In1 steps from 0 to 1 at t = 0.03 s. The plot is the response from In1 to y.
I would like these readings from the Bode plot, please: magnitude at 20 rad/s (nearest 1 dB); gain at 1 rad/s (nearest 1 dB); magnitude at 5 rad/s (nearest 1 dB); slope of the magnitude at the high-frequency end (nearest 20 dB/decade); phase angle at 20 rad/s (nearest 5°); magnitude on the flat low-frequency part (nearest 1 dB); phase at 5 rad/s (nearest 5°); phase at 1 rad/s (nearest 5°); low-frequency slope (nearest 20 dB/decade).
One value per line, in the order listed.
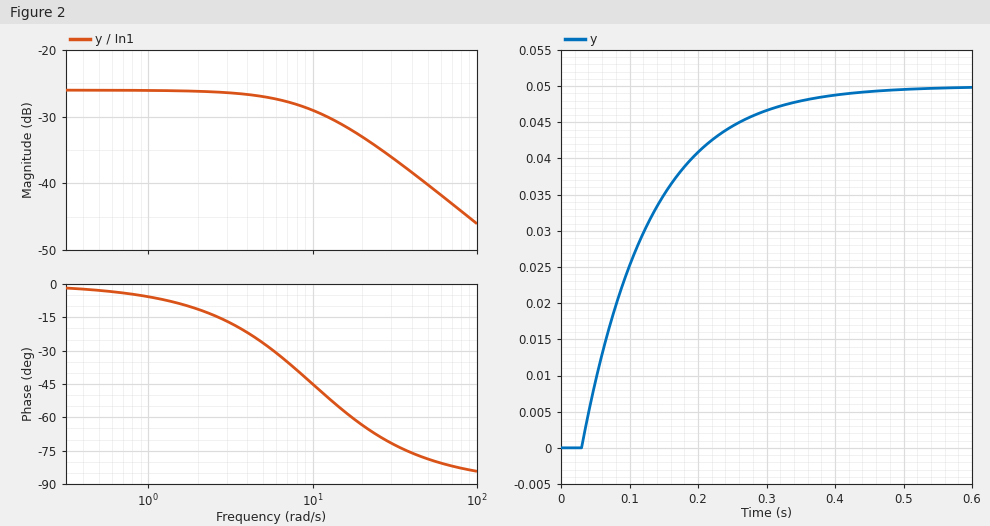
-33 dB
-26 dB
-27 dB
-20 dB/decade
-65°
-26 dB
-25°
-5°
0 dB/decade
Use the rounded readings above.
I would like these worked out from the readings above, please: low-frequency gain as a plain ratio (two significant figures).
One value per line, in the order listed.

0.050
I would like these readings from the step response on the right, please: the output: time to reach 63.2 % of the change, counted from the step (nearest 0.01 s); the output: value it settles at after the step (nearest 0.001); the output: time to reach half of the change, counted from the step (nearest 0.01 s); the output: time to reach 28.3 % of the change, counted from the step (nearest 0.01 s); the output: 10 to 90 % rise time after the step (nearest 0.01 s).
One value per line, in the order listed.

0.10 s
0.050
0.07 s
0.03 s
0.22 s
